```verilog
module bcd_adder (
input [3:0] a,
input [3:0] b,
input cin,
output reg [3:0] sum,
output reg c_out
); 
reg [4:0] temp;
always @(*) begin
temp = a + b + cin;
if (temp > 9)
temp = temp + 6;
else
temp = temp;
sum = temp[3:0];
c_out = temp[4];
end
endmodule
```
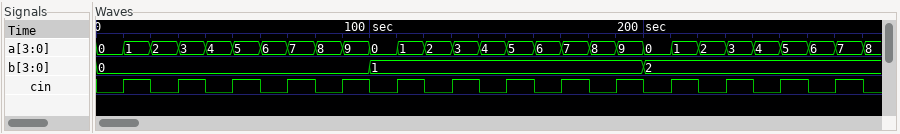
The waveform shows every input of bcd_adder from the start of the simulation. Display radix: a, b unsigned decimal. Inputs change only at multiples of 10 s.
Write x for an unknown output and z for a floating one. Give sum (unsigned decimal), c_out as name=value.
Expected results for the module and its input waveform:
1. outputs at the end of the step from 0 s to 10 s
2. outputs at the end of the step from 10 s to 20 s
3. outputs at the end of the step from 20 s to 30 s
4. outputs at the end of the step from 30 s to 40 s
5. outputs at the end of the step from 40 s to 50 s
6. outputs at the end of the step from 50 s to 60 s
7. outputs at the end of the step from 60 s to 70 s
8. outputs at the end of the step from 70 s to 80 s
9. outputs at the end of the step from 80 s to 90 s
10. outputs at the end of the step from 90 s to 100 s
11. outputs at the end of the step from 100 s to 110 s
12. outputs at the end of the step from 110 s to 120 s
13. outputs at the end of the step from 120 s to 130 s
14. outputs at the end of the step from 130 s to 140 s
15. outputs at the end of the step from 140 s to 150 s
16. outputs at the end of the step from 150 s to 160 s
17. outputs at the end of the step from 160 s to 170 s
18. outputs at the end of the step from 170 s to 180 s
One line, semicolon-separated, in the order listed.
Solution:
sum=0, c_out=0; sum=2, c_out=0; sum=2, c_out=0; sum=4, c_out=0; sum=4, c_out=0; sum=6, c_out=0; sum=6, c_out=0; sum=8, c_out=0; sum=8, c_out=0; sum=0, c_out=1; sum=1, c_out=0; sum=3, c_out=0; sum=3, c_out=0; sum=5, c_out=0; sum=5, c_out=0; sum=7, c_out=0; sum=7, c_out=0; sum=9, c_out=0
